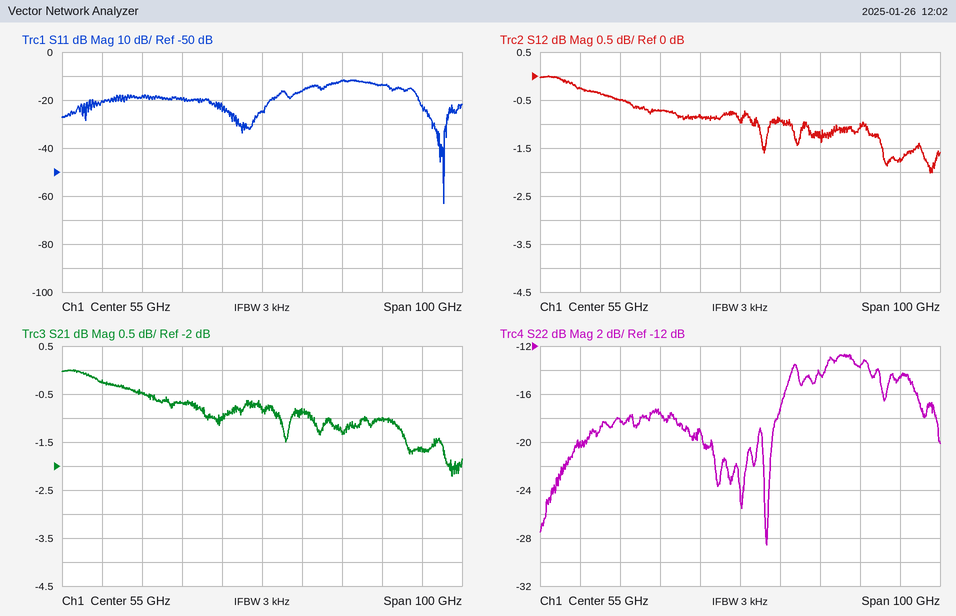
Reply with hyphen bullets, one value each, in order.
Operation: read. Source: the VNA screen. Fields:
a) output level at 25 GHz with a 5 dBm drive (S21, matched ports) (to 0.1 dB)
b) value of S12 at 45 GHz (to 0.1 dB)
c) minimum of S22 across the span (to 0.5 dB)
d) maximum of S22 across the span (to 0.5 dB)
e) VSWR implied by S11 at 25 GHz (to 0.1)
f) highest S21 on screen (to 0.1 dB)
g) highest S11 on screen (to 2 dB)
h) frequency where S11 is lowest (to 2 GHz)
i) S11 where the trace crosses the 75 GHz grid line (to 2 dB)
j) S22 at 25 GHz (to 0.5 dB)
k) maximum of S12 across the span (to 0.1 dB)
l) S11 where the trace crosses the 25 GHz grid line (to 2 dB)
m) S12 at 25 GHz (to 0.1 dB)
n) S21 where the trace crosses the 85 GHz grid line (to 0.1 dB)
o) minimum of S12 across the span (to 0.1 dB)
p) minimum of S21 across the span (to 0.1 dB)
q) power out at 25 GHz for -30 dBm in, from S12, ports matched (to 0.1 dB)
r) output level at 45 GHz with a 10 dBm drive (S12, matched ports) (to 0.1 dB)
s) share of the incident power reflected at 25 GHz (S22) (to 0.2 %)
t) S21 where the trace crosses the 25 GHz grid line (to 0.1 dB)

- 4.5 dBm
- -0.8 dB
- -28.5 dB
- -12.5 dB
- 1.3
- 0.0 dB
- -12 dB
- 100 GHz
- -12 dB
- -18.0 dB
- 0.0 dB
- -18 dB
- -0.5 dB
- -1.0 dB
- -2.0 dB
- -2.2 dB
- -30.5 dBm
- 9.2 dBm
- 1.6 %
- -0.5 dB
